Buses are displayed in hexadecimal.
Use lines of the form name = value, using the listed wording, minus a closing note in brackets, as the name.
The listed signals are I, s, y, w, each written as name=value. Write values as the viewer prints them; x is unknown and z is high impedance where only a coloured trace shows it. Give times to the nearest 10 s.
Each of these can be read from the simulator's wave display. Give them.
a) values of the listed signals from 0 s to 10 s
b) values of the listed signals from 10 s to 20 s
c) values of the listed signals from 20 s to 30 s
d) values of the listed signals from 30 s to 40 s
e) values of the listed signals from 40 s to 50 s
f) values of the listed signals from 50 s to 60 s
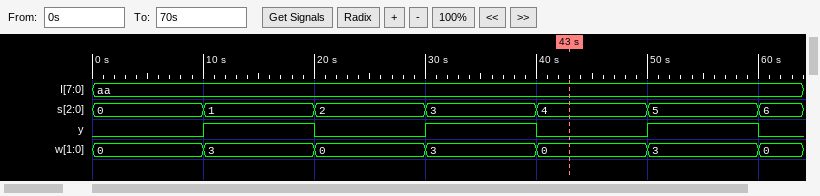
values of the listed signals from 0 s to 10 s = I=aa, s=0, y=0, w=0
values of the listed signals from 10 s to 20 s = I=aa, s=1, y=1, w=3
values of the listed signals from 20 s to 30 s = I=aa, s=2, y=0, w=0
values of the listed signals from 30 s to 40 s = I=aa, s=3, y=1, w=3
values of the listed signals from 40 s to 50 s = I=aa, s=4, y=0, w=0
values of the listed signals from 50 s to 60 s = I=aa, s=5, y=1, w=3
